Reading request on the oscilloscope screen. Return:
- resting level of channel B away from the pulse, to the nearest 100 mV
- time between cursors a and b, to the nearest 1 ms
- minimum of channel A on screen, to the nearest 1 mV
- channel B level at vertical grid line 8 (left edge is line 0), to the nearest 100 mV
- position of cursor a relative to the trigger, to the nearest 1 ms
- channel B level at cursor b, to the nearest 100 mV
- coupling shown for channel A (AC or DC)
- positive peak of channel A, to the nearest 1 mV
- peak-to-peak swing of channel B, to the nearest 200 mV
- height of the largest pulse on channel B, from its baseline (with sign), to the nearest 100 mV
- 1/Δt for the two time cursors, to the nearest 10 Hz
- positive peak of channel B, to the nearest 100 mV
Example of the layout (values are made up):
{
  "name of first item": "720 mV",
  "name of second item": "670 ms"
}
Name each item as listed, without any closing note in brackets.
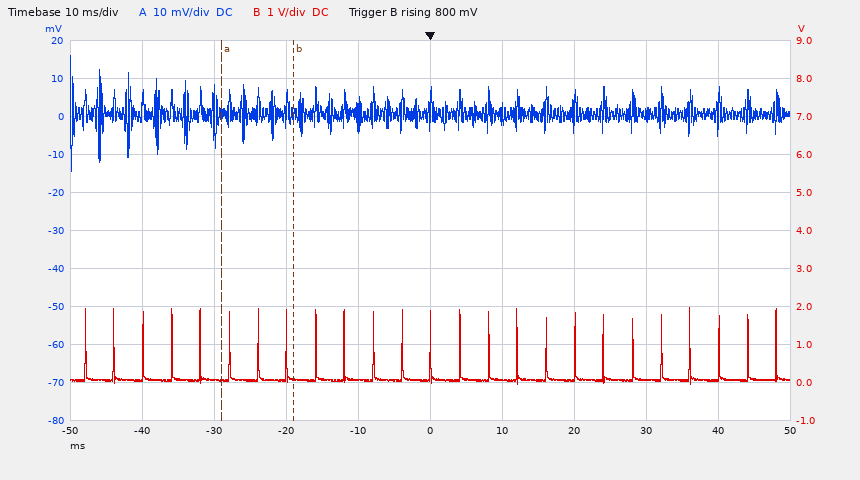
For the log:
{
  "resting level of channel B away from the pulse, to the nearest 100 mV": "100 mV",
  "time between cursors a and b, to the nearest 1 ms": "10 ms",
  "minimum of channel A on screen, to the nearest 1 mV": "-14 mV",
  "channel B level at vertical grid line 8 (left edge is line 0), to the nearest 100 mV": "100 mV",
  "position of cursor a relative to the trigger, to the nearest 1 ms": "-29 ms",
  "channel B level at cursor b, to the nearest 100 mV": "100 mV",
  "coupling shown for channel A": "DC",
  "positive peak of channel A, to the nearest 1 mV": "16 mV",
  "peak-to-peak swing of channel B, to the nearest 200 mV": "2.0 V",
  "height of the largest pulse on channel B, from its baseline (with sign), to the nearest 100 mV": "+1.9 V",
  "1/Δt for the two time cursors, to the nearest 10 Hz": "100 Hz",
  "positive peak of channel B, to the nearest 100 mV": "2.0 V"
}
